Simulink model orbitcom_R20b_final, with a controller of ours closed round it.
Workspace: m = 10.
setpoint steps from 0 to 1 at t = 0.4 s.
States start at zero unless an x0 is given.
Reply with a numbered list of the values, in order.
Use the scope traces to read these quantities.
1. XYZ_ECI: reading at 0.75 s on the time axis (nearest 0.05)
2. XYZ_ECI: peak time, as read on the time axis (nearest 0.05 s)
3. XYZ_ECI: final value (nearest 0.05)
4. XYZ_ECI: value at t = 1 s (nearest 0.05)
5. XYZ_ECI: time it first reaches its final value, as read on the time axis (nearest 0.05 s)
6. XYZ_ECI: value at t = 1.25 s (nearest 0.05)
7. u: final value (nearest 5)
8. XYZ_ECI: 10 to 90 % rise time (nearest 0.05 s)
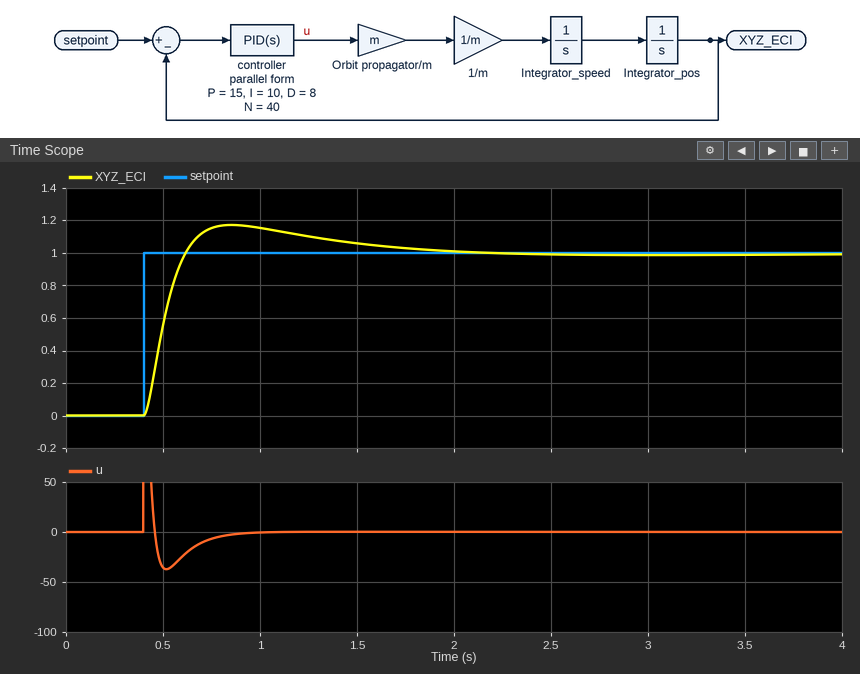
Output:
1. 1.15
2. 0.85 s
3. 1.00
4. 1.15
5. 0.60 s
6. 1.10
7. 0
8. 0.15 s
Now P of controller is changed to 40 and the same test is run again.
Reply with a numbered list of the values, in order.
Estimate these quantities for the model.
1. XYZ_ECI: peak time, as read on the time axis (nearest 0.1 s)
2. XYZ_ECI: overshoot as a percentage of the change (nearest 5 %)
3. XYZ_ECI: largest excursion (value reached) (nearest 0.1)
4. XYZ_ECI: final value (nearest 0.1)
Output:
1. 0.7 s
2. 30 %
3. 1.3
4. 1.0
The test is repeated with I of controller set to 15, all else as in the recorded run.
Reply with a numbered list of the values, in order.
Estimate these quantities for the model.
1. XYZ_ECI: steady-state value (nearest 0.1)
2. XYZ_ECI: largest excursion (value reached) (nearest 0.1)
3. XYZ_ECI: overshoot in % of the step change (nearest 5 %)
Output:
1. 1.0
2. 1.2
3. 20 %
